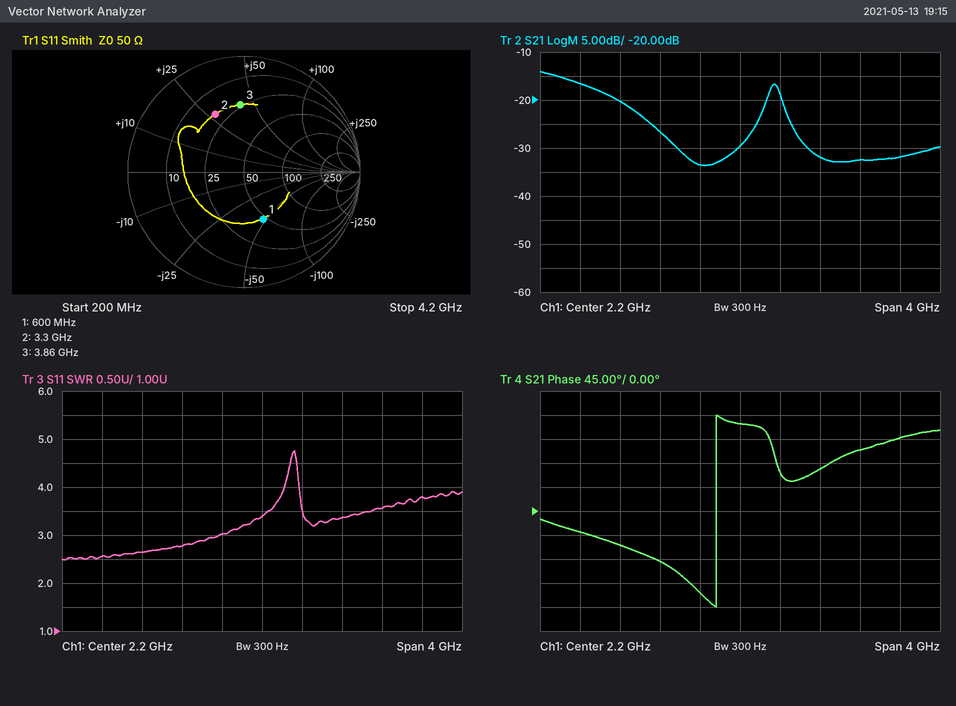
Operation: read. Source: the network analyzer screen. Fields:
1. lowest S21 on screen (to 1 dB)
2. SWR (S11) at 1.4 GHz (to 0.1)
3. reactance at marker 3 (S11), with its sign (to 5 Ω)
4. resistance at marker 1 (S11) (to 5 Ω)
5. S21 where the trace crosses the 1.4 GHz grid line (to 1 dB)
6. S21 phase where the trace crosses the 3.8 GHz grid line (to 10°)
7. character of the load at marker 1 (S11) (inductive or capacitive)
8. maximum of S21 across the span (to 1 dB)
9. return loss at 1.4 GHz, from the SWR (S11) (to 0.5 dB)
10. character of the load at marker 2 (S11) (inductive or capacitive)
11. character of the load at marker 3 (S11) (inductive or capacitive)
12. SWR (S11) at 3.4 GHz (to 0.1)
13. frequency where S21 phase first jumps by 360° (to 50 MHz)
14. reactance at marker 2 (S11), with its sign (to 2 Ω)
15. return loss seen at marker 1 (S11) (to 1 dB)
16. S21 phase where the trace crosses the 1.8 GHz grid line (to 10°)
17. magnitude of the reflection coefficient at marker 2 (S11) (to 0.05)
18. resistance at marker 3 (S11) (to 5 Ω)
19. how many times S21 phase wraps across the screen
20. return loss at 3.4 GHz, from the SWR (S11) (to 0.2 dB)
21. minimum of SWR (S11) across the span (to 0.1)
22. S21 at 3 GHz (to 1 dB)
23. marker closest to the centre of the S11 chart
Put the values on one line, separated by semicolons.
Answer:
-34 dB; 2.8; +40 Ω; 45 Ω; -27 dB; 140°; capacitive; -14 dB; 6.5 dB; inductive; inductive; 3.6; 1.95 GHz; +28 Ω; 7 dB; -150°; 0.55; 25 Ω; 1; 5.0 dB; 2.5; -32 dB; marker 1
